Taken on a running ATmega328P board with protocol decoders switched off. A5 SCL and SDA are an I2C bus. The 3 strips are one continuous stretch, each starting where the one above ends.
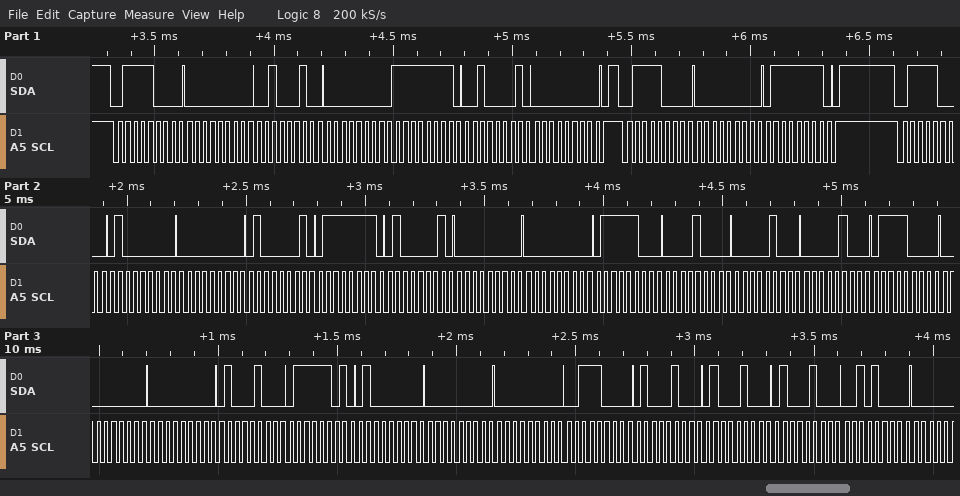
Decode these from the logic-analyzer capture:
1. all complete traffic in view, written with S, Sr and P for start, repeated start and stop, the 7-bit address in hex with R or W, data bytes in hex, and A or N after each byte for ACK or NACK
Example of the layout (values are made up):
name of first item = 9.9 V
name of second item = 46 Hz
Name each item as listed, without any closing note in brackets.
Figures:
all complete traffic in view, written with S, Sr and P for start, repeated start and stop, the 7-bit address in hex with R or W, data bytes in hex, and A or N after each byte for ACK or NACK = S 3CW A 00 A 22 A 00 A FF A 21 A 00 A P S 3CW A 00 A 7F A P S 3CW A 40 A 00 A 41 A 7F A 41 A 00 A 00 A 7C A 08 A 04 A 04 A 78 A 00 A 00 A 44 A 7D A 40 A 00 A 00 A 38 A 44 A 44 A 44 A 28 A
